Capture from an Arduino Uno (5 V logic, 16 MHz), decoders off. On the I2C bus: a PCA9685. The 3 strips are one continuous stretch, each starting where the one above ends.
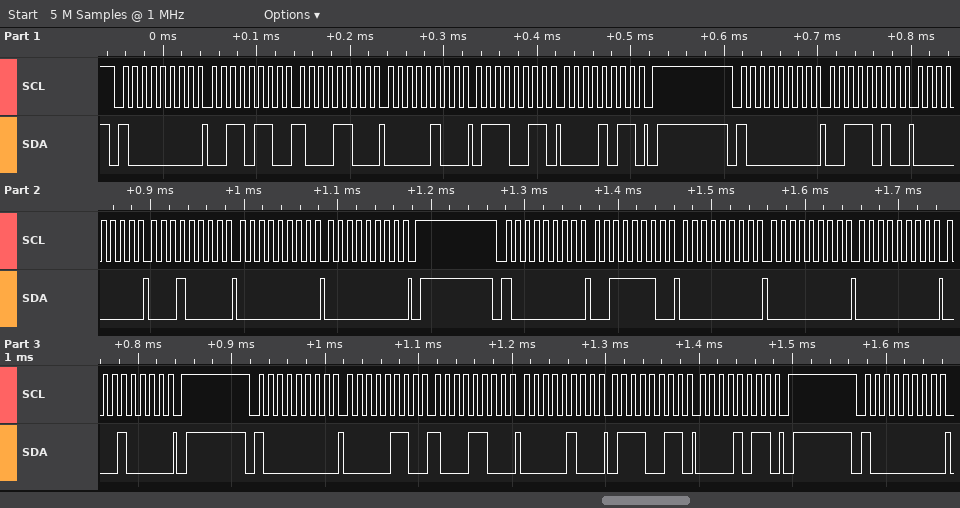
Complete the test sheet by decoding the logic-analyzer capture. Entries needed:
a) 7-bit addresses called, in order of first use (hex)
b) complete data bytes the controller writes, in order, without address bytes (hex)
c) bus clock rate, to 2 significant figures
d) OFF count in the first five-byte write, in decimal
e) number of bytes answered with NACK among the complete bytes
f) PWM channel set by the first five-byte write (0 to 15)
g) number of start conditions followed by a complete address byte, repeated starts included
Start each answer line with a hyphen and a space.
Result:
- 0x40
- 36 8C 04 73 0B 3A 00 10 00 00 3E 00 00 00 10 06 8C 04 73 0B
- 100 kHz
- 2931
- 0
- 12
- 5
